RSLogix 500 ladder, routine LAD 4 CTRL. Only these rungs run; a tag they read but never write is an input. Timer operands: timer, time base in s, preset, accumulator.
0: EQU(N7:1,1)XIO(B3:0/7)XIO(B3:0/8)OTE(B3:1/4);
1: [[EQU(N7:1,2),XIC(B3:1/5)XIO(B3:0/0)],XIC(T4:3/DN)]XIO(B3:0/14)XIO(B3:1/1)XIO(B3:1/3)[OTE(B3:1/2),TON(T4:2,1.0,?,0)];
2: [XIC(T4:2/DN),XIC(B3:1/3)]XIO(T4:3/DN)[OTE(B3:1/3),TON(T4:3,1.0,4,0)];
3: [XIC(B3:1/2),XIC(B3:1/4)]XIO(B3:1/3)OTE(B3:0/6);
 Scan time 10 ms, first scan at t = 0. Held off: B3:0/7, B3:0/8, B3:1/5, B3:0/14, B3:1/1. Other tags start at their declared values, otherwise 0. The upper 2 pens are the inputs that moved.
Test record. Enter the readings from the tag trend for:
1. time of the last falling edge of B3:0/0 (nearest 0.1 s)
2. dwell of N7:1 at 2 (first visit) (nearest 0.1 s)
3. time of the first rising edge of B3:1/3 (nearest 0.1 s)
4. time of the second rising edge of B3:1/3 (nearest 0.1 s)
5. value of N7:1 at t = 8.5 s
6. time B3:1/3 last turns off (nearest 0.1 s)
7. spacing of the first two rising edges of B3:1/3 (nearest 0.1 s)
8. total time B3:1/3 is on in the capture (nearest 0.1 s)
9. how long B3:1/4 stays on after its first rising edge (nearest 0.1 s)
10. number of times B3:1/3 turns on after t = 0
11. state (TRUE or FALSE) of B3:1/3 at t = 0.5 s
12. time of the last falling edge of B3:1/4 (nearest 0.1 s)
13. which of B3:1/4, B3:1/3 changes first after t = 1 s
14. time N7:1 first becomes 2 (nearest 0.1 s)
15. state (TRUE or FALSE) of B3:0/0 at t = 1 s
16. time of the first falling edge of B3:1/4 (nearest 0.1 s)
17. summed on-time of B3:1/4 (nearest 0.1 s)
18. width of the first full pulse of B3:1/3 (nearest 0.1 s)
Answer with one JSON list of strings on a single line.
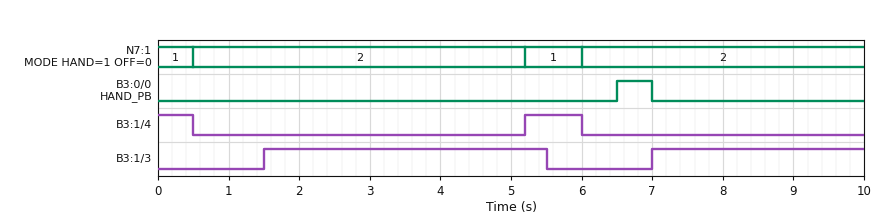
["7.0 s", "4.7 s", "1.5 s", "7.0 s", "2", "5.5 s", "5.5 s", "7.0 s", "0.8 s", "2", "FALSE", "6.0 s", "B3:1/3", "0.5 s", "FALSE", "0.5 s", "1.3 s", "4.0 s"]
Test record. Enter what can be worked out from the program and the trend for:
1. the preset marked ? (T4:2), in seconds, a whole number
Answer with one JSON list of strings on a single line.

["1 s"]
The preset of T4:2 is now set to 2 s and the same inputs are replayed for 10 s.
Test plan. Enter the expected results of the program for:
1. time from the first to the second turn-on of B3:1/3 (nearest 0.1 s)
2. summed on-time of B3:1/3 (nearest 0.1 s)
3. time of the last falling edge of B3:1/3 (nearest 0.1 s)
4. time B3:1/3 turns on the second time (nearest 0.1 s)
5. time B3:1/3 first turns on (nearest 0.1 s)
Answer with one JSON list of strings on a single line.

["6.0 s", "5.5 s", "6.5 s", "8.5 s", "2.5 s"]
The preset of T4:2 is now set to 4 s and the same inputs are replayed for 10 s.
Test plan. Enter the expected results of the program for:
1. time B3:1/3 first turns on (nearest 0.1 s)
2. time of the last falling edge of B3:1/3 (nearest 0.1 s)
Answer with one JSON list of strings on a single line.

["4.5 s", "8.5 s"]
